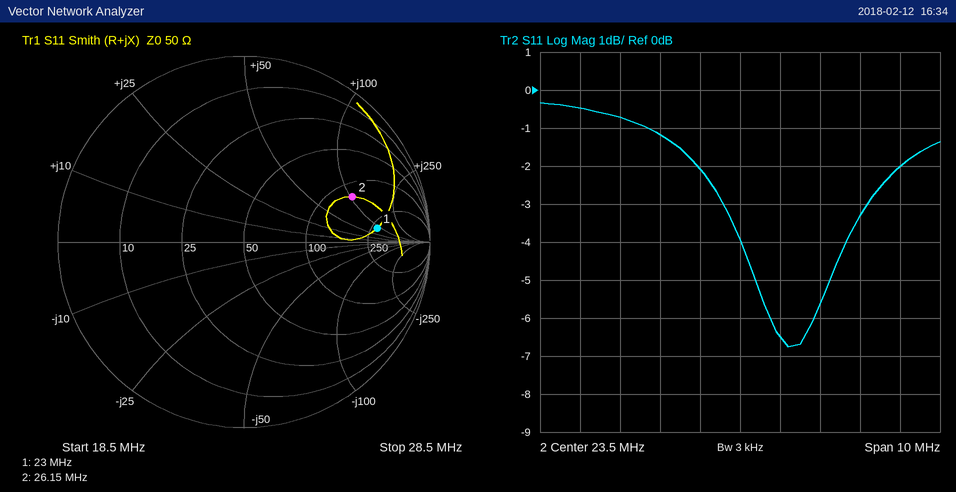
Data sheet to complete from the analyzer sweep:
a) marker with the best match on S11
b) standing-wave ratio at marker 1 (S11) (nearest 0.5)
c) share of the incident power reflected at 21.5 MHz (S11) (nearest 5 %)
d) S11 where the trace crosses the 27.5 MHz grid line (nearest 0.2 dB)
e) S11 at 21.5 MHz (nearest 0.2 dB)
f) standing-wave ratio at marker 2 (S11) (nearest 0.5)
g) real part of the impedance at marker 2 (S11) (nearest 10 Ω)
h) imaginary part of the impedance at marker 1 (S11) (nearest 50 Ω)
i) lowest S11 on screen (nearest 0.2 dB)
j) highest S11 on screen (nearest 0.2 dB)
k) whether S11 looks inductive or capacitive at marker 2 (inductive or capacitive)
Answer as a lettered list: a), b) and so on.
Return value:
a) marker 2
b) 6.0
c) 75 %
d) -2.0 dB
e) -1.2 dB
f) 4.5
g) 130 Ω
h) +100 Ω
i) -6.8 dB
j) -0.4 dB
k) inductive
